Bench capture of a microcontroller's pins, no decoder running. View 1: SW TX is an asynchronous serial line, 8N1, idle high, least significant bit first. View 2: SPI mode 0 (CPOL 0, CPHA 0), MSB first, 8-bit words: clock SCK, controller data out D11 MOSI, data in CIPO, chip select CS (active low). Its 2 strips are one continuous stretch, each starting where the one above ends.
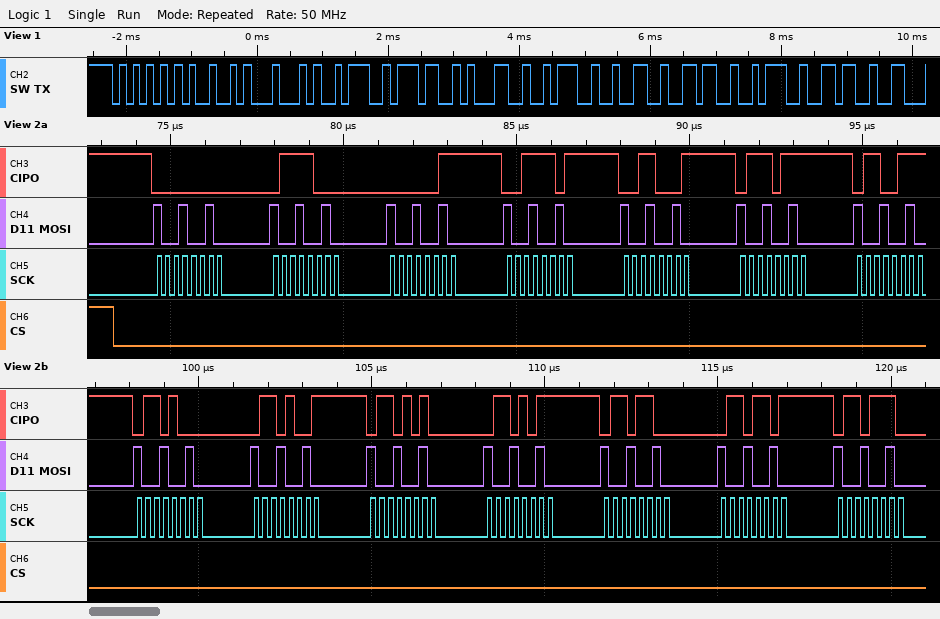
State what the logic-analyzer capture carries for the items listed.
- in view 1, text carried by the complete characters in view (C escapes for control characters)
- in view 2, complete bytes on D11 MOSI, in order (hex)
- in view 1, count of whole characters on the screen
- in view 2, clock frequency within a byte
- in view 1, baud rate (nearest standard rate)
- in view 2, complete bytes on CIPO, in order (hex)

"UID:71:26:6"
0x92 0x92 0x92 0x92 0x92 0x92 0x92 0x92 0x92 0x92 0x92 0x92 0x92 0x92
11
4 MHz
9600 baud
0x00 0x78 0x03 0x3D 0x31 0x77 0x67 0x68 0x69 0x6A 0x6B 0x6C 0x6D 0x6E
